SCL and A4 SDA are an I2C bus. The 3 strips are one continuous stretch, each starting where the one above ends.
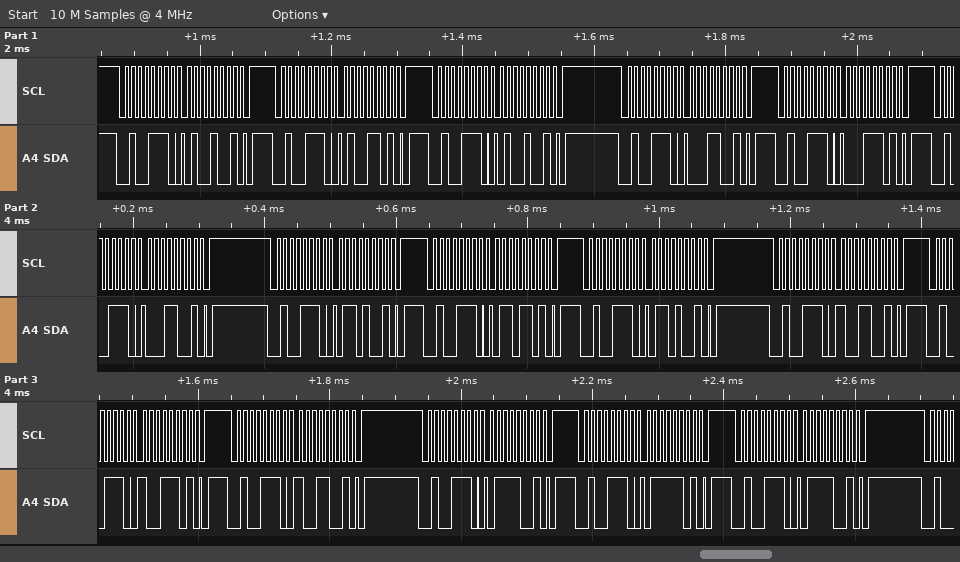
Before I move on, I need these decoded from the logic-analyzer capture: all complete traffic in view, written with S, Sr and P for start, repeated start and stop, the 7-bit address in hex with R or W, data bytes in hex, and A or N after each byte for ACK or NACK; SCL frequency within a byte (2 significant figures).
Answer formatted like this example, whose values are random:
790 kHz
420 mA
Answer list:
S 27W A 49 A P S 27W A 4D A P S 27W A 49 A P S 27W A 19 A P S 27W A 1D A P S 27W A 19 A P S 27W A 69 A P S 27W A 6D A P S 27W A 69 A P S 27W A 99 A P S 27W A 9D A P S 27W A 99 A P S 27W A 79 A P S 27W A 7D A P S 27W A 79 A P
100 kHz
